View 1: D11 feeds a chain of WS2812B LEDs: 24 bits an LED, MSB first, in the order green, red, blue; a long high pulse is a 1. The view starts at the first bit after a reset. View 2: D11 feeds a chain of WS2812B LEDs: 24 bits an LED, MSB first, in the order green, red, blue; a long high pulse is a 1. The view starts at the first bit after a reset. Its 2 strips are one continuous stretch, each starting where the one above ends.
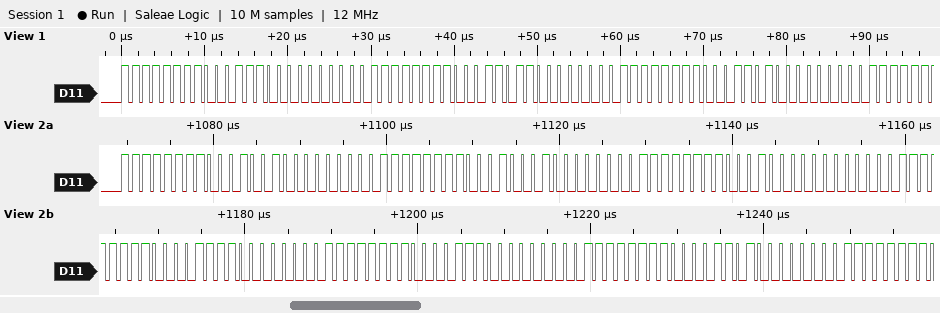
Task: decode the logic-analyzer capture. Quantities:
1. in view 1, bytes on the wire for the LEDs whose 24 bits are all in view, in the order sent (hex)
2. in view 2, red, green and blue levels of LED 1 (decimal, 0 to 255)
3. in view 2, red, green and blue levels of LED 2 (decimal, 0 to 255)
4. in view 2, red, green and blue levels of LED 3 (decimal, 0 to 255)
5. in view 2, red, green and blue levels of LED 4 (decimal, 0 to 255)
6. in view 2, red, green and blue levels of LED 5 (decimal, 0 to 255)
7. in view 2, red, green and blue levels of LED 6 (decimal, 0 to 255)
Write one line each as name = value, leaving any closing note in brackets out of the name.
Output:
in view 1, bytes on the wire for the LEDs whose 24 bits are all in view, in the order sent = FF 1C 00 FF 1B 00 FF 1A 00
in view 2, red, green and blue levels of LED 1 = 18, 255, 0
in view 2, red, green and blue levels of LED 2 = 17, 255, 0
in view 2, red, green and blue levels of LED 3 = 16, 255, 0
in view 2, red, green and blue levels of LED 4 = 15, 255, 0
in view 2, red, green and blue levels of LED 5 = 14, 255, 0
in view 2, red, green and blue levels of LED 6 = 13, 255, 0
